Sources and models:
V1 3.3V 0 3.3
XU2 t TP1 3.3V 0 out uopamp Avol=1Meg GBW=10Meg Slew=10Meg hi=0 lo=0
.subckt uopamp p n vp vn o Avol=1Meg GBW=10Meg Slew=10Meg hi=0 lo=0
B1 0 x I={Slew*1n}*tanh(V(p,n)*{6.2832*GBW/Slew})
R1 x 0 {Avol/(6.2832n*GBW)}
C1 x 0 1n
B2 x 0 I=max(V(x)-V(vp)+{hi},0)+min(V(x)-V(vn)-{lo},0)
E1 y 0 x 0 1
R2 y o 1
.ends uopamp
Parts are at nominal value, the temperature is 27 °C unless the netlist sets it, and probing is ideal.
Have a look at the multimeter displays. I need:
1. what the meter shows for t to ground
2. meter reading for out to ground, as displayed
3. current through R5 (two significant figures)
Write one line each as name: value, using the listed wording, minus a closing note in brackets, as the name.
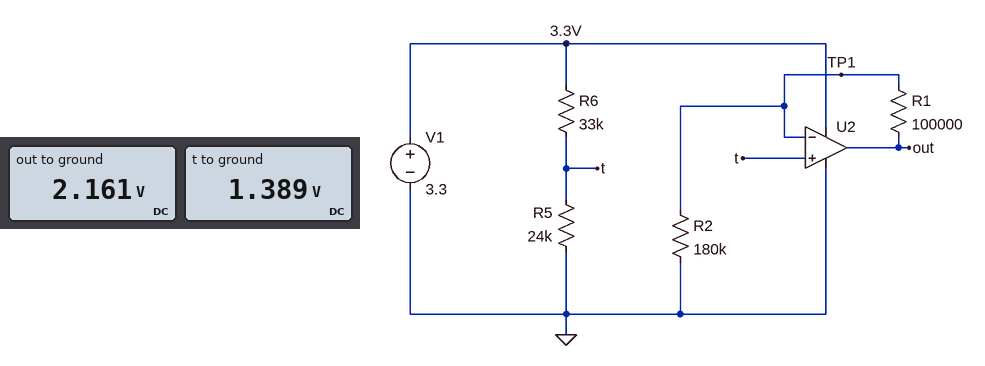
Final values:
what the meter shows for t to ground: 1.389 V
meter reading for out to ground, as displayed: 2.161 V
current through R5: 58 µA
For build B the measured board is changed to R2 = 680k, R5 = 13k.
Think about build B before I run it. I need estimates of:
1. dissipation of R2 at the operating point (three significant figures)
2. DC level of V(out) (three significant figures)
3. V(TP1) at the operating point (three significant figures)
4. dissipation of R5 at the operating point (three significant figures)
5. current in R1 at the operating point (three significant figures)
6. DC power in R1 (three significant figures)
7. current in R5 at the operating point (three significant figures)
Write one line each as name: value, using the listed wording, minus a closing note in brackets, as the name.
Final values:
dissipation of R2 at the operating point: 1.28 µW
DC level of V(out): 1.07 V
V(TP1) at the operating point: 933 mV
dissipation of R5 at the operating point: 66.9 µW
current in R1 at the operating point: 1.37 µA
DC power in R1: 188 nW
current in R5 at the operating point: 71.7 µA
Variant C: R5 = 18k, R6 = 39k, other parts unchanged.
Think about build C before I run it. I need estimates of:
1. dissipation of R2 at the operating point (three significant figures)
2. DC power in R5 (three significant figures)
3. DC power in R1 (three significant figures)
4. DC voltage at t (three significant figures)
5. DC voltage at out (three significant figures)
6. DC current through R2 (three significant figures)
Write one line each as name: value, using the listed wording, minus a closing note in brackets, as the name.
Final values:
dissipation of R2 at the operating point: 6.03 µW
DC power in R5: 60.3 µW
DC power in R1: 3.35 µW
DC voltage at t: 1.04 V
DC voltage at out: 1.62 V
DC current through R2: 5.79 µA
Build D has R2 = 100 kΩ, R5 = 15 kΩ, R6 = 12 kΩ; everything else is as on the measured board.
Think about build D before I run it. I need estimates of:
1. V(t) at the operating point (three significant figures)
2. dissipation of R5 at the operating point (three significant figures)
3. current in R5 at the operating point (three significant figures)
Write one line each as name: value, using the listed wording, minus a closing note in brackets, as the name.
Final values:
V(t) at the operating point: 1.83 V
dissipation of R5 at the operating point: 224 µW
current in R5 at the operating point: 122 µA
